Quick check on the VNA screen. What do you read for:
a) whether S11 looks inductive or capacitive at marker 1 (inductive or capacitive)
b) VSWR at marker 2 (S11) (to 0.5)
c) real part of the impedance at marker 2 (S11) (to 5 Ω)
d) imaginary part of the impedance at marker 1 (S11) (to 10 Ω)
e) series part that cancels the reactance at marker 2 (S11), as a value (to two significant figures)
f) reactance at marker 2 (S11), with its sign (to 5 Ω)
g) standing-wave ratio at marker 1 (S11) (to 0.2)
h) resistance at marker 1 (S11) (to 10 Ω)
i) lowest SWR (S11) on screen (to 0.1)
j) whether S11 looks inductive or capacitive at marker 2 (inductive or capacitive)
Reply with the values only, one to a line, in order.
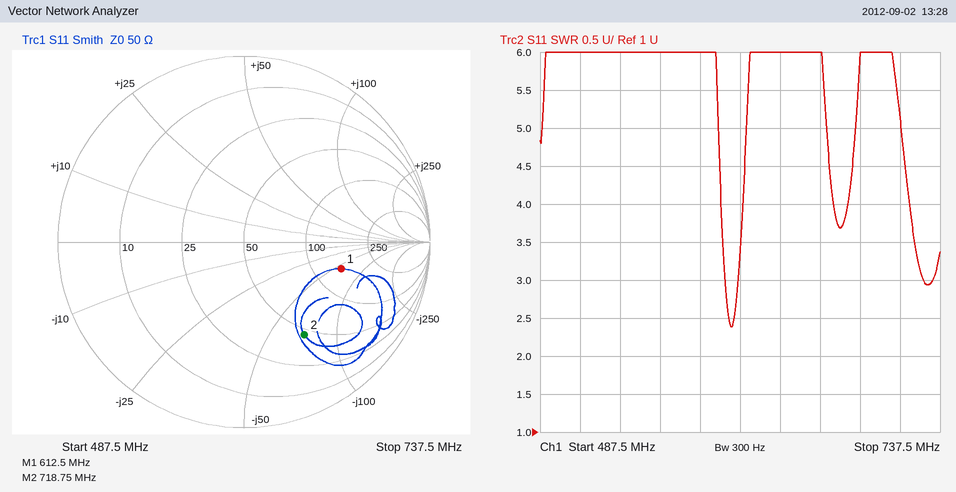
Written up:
capacitive
4.0
45 Ω
-60 Ω
16 nH
-70 Ω
3.4
140 Ω
2.4
capacitive
